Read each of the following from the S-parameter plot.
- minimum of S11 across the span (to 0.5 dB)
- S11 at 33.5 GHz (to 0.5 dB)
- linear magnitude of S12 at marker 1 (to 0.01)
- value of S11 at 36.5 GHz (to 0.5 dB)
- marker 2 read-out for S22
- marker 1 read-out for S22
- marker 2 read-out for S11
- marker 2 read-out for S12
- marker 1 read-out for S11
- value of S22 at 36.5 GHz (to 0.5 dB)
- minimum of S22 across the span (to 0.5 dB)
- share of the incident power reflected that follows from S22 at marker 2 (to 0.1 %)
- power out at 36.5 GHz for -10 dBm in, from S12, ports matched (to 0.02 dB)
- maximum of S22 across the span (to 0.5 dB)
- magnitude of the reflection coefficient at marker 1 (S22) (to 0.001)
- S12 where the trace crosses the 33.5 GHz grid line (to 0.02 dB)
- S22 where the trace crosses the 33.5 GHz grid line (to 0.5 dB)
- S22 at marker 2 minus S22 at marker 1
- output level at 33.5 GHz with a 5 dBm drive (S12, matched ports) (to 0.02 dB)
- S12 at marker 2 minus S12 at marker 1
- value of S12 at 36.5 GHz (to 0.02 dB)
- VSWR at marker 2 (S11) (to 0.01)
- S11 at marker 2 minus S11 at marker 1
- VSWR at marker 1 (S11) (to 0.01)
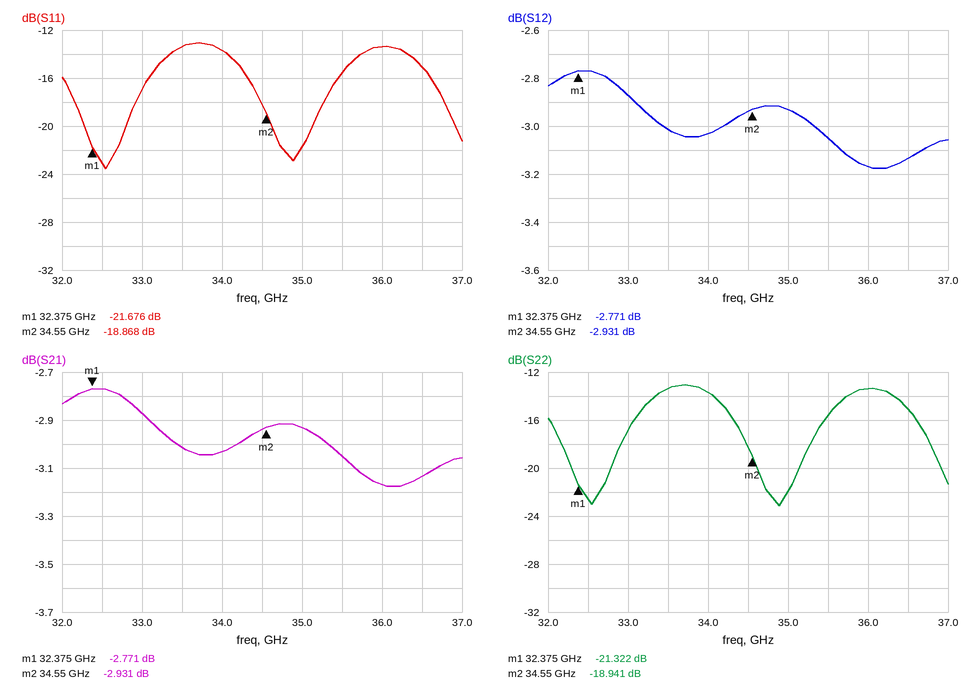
-23.5 dB
-13.5 dB
0.73
-15.0 dB
-18.941 dB
-21.322 dB
-18.868 dB
-2.931 dB
-21.676 dB
-15.0 dB
-23.0 dB
1.3 %
-13.14 dBm
-13.0 dB
0.086
-3.02 dB
-13.5 dB
2.381 dB
1.98 dBm
-0.160 dB
-3.14 dB
1.26
2.808 dB
1.18
